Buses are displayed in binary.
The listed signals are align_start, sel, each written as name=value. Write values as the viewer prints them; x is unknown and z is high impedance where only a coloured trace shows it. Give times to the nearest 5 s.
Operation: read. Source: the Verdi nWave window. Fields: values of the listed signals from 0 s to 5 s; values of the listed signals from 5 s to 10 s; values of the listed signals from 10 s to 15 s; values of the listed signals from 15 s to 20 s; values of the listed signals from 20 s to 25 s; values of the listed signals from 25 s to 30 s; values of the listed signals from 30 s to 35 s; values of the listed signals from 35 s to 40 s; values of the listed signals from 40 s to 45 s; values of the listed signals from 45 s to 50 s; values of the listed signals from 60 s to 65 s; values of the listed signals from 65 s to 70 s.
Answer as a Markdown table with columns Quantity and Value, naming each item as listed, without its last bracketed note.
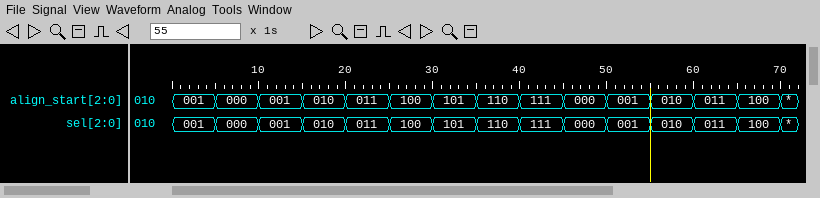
| Quantity | Value |
|---|---|
| values of the listed signals from 0 s to 5 s | align_start=001, sel=001 |
| values of the listed signals from 5 s to 10 s | align_start=000, sel=000 |
| values of the listed signals from 10 s to 15 s | align_start=001, sel=001 |
| values of the listed signals from 15 s to 20 s | align_start=010, sel=010 |
| values of the listed signals from 20 s to 25 s | align_start=011, sel=011 |
| values of the listed signals from 25 s to 30 s | align_start=100, sel=100 |
| values of the listed signals from 30 s to 35 s | align_start=101, sel=101 |
| values of the listed signals from 35 s to 40 s | align_start=110, sel=110 |
| values of the listed signals from 40 s to 45 s | align_start=111, sel=111 |
| values of the listed signals from 45 s to 50 s | align_start=000, sel=000 |
| values of the listed signals from 60 s to 65 s | align_start=011, sel=011 |
| values of the listed signals from 65 s to 70 s | align_start=100, sel=100 |
